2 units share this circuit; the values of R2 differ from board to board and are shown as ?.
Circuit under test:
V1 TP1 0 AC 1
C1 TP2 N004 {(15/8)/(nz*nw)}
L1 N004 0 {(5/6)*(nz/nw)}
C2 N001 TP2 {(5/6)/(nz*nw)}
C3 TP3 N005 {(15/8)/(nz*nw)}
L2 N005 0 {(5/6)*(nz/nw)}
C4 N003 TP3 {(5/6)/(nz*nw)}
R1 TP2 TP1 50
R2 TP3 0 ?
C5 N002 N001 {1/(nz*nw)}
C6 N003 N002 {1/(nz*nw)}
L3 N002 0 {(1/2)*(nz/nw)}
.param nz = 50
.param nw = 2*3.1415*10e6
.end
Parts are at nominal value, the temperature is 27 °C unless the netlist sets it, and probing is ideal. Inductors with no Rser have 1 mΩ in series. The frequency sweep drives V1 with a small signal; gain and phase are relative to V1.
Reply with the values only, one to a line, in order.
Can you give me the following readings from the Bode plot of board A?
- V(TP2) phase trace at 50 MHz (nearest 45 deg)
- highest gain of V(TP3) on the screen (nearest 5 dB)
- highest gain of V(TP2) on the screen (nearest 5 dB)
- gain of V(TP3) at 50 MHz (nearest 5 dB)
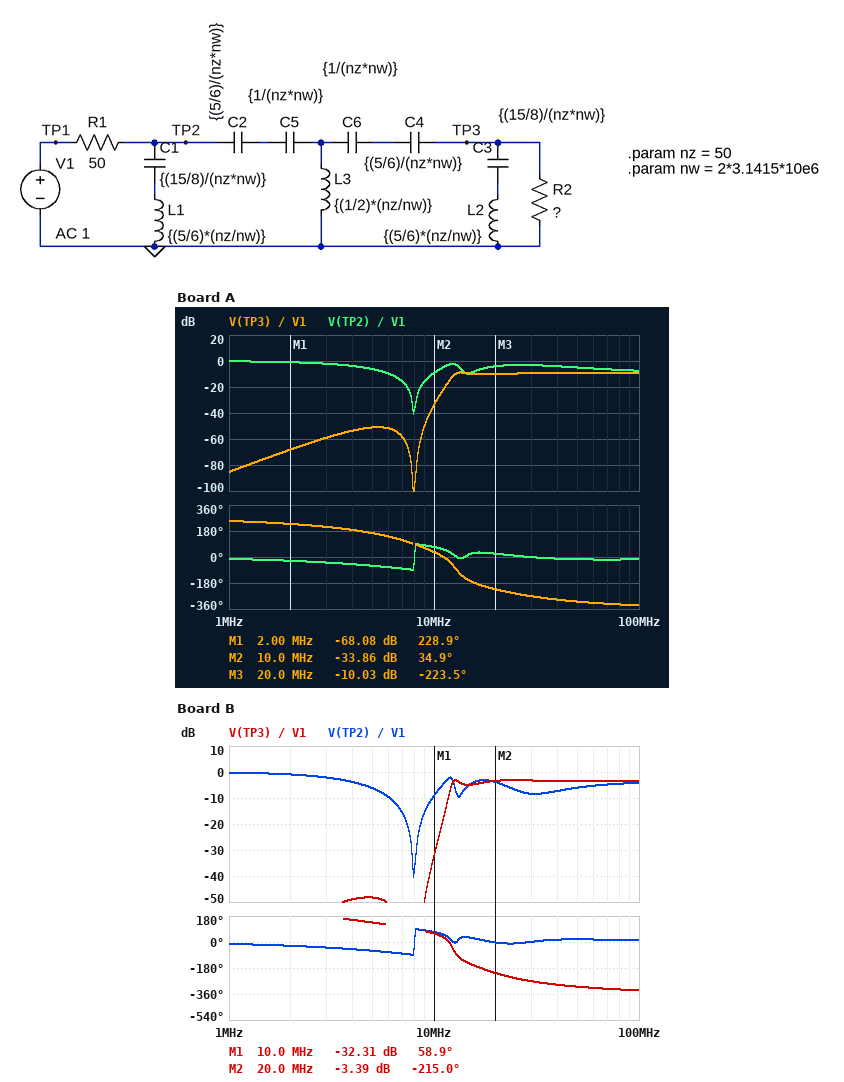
0 deg
-10 dB
0 dB
-10 dB
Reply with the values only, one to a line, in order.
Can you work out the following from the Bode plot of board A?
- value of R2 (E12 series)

27 Ω
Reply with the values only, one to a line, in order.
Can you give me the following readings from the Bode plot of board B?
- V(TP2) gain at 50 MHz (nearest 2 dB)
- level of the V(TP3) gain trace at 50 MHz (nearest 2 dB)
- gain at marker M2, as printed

-6 dB
-4 dB
-3.39 dB
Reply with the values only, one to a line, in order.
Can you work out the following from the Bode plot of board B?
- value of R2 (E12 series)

100 Ω
